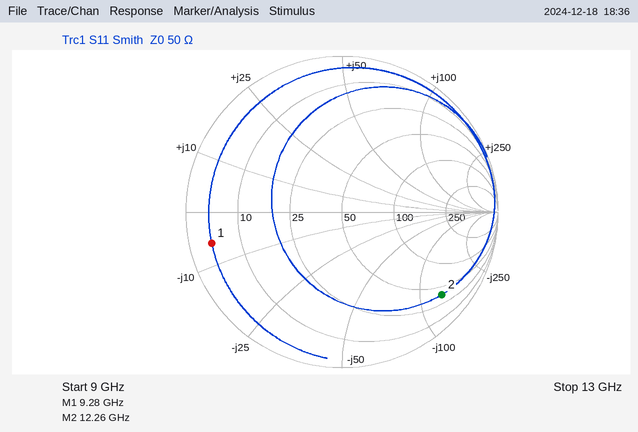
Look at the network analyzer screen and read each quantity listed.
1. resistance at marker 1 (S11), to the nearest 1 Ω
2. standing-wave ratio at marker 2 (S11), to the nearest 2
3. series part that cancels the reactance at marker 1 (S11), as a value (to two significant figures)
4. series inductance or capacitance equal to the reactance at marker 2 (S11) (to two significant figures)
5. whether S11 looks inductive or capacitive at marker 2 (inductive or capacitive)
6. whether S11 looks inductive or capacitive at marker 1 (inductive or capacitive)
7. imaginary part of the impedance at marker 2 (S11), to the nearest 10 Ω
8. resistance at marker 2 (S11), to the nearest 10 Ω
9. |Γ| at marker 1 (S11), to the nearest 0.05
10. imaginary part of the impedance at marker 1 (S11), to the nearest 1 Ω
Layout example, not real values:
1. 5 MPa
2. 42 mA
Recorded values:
1. 4 Ω
2. 10
3. 100 pH
4. 100 fF
5. capacitive
6. capacitive
7. -130 Ω
8. 40 Ω
9. 0.85
10. -6 Ω
